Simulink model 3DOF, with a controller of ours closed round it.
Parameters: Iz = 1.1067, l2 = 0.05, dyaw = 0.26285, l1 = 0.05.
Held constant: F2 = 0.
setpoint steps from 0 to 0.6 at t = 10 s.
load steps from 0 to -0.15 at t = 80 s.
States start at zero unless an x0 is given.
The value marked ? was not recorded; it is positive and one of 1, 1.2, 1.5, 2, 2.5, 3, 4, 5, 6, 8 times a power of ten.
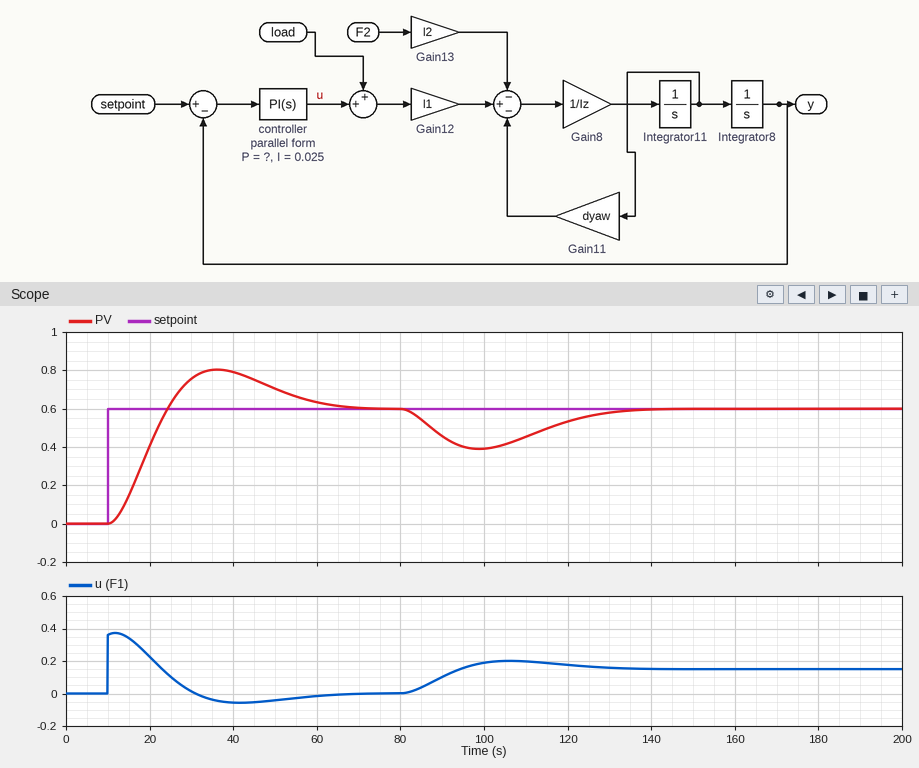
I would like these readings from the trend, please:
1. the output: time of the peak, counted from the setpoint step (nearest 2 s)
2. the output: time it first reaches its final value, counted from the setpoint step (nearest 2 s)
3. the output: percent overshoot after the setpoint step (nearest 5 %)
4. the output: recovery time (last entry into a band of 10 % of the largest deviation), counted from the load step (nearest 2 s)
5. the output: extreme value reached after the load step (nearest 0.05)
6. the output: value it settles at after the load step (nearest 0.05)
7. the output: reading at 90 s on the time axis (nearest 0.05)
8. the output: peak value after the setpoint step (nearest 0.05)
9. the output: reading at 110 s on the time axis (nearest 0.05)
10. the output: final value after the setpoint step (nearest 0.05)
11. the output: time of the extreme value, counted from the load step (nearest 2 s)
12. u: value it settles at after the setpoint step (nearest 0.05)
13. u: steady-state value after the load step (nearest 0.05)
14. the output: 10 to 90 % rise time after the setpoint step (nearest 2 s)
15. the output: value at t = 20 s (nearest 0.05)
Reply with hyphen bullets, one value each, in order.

- 26 s
- 14 s
- 35 %
- 50 s
- 0.40
- 0.60
- 0.45
- 0.80
- 0.45
- 0.60
- 18 s
- 0.00
- 0.15
- 10 s
- 0.40
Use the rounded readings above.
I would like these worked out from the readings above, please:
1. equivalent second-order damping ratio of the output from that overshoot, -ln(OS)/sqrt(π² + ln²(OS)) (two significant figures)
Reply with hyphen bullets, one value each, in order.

- 0.32
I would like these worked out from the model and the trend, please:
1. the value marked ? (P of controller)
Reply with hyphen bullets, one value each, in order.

- 0.6
